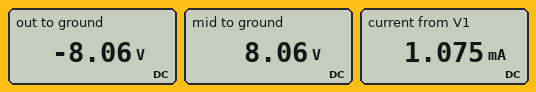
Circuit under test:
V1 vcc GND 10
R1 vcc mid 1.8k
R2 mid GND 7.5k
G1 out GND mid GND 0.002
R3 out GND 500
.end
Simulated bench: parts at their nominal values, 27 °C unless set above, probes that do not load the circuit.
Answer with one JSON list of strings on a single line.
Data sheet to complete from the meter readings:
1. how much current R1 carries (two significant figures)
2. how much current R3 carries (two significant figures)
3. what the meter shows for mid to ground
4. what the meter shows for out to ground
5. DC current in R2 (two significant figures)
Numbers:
["1.1 mA", "16 mA", "8.06 V", "-8.06 V", "1.1 mA"]
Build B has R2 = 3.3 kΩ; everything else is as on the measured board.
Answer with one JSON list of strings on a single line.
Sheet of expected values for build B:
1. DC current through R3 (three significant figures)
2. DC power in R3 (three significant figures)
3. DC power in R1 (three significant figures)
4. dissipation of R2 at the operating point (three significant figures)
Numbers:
["12.9 mA", "83.7 mW", "6.92 mW", "12.7 mW"]
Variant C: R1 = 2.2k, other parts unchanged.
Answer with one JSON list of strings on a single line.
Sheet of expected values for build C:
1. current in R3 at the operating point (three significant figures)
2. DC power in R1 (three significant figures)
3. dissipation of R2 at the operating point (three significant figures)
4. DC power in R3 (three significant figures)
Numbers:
["15.5 mA", "2.34 mW", "7.97 mW", "120 mW"]
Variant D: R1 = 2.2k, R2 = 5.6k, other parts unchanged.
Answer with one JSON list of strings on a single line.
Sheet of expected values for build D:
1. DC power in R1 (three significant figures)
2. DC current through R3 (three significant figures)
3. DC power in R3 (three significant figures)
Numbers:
["3.62 mW", "14.4 mA", "103 mW"]
